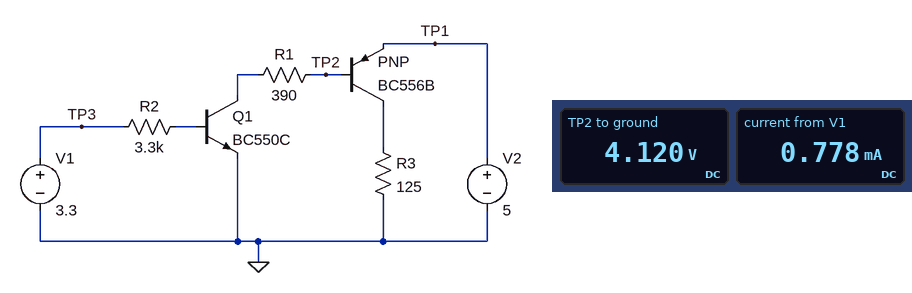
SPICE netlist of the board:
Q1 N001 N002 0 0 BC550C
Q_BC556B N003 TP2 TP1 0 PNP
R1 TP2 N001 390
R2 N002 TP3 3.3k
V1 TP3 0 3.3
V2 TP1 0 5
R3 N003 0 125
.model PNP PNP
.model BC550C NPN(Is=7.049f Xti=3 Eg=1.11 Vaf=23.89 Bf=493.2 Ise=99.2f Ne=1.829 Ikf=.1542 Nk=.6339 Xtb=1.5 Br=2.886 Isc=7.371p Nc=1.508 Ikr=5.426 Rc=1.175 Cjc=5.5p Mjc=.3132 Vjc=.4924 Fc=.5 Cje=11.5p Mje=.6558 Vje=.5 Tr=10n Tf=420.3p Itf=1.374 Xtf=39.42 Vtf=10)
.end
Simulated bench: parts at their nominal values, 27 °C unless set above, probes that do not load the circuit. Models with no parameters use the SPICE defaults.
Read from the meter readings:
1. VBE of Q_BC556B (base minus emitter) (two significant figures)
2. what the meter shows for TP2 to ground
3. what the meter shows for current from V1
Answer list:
-880 mV
4.120 V
0.778 mA
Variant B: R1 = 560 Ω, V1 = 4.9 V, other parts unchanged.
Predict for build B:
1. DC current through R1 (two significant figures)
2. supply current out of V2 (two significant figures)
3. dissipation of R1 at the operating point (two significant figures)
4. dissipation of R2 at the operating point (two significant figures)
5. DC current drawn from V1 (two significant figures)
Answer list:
7.3 mA
47 mA
30 mW
5.3 mW
1.3 mA
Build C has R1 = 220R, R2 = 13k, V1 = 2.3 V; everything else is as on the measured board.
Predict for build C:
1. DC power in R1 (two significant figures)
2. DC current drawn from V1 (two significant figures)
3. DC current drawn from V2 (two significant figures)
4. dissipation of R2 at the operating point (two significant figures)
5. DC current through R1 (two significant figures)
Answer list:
71 mW
120 µA
58 mA
190 µW
18 mA
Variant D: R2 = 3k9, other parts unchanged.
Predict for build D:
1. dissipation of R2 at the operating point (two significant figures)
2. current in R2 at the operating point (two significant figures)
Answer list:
1.7 mW
660 µA
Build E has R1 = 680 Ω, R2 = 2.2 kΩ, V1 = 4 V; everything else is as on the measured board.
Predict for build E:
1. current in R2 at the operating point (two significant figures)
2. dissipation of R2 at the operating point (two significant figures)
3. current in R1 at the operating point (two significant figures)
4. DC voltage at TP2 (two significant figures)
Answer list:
1.5 mA
4.9 mW
6.0 mA
4.1 V
